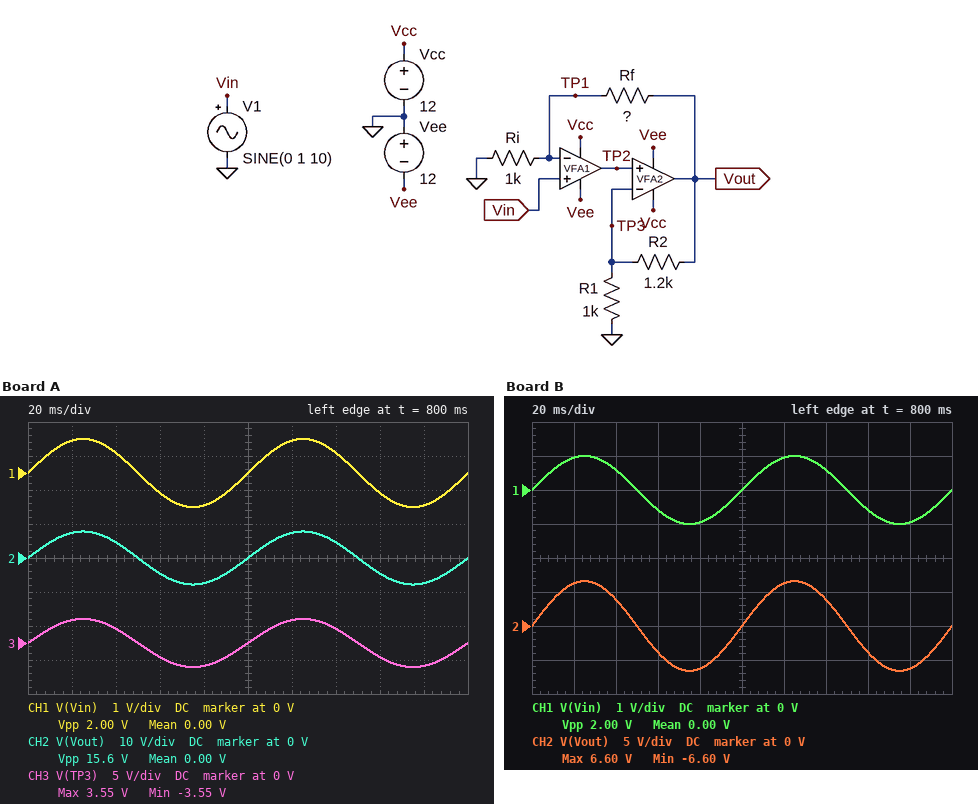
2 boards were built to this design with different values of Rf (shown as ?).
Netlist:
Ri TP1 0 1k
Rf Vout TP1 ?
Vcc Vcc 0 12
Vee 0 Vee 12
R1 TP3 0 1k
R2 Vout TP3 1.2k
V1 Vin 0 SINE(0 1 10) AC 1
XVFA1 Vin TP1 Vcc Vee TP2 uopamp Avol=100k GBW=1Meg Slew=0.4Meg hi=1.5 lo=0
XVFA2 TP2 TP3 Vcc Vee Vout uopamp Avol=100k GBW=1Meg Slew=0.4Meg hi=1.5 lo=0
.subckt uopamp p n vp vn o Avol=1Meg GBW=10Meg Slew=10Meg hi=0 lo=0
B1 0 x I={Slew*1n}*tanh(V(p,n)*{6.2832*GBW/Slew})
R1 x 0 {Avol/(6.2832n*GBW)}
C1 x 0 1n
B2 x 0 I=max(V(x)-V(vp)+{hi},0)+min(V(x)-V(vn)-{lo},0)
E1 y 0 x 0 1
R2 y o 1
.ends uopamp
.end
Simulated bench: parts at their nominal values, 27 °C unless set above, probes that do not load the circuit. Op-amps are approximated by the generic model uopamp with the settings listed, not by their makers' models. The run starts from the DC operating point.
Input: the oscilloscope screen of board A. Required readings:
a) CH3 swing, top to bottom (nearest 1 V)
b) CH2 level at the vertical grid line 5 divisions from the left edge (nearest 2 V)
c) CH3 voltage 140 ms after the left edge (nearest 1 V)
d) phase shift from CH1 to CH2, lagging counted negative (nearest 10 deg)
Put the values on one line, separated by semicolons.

7 V; 0 V; 2 V; 0 deg
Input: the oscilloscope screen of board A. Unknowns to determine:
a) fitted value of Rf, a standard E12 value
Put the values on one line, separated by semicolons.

6.8 kΩ
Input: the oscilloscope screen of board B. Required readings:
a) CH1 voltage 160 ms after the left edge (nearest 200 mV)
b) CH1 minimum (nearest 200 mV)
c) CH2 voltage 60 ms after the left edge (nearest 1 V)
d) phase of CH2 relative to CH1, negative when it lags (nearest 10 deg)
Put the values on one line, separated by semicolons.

-600 mV; -1.0 V; -4 V; 0 deg
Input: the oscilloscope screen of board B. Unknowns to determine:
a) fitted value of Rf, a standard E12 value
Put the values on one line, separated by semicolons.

5.6 kΩ
